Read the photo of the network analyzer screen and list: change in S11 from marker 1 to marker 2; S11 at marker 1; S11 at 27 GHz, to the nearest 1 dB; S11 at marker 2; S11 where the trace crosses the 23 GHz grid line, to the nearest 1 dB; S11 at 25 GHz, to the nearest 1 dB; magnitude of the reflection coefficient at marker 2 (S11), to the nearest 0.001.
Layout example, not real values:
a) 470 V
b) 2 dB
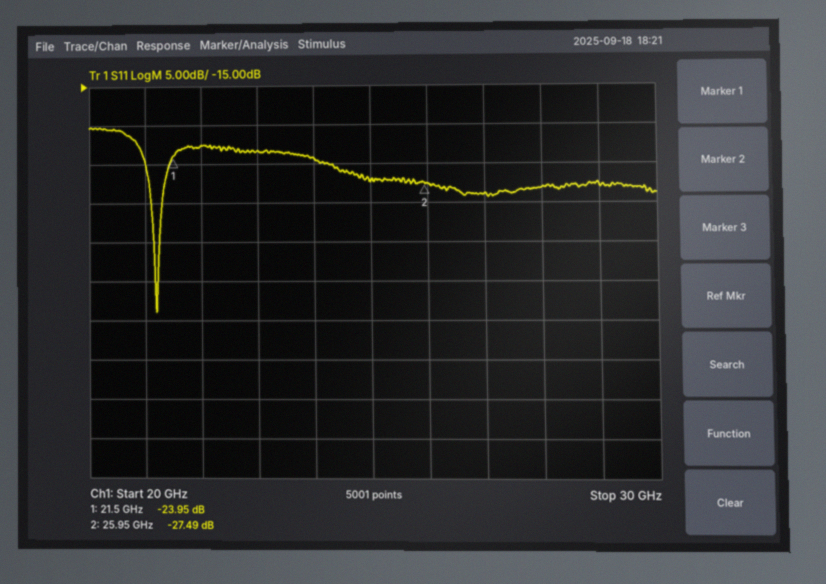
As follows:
a) -3.54 dB
b) -23.95 dB
c) -29 dB
d) -27.49 dB
e) -23 dB
f) -27 dB
g) 0.042
